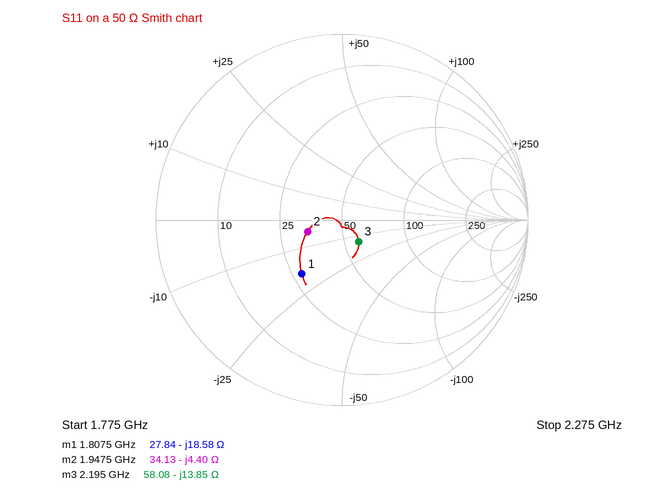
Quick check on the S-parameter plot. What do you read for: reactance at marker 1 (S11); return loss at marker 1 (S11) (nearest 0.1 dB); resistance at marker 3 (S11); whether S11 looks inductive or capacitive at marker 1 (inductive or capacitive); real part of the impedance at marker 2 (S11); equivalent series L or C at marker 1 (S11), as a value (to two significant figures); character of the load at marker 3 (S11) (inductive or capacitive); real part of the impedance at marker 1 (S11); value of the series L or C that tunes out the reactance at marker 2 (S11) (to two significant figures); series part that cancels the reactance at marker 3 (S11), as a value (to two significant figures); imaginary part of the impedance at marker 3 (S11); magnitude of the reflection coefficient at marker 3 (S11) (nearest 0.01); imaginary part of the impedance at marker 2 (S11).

-18.58 Ω
8.8 dB
58.08 Ω
capacitive
34.13 Ω
4.7 pF
capacitive
27.84 Ω
360 pH
1.0 nH
-13.85 Ω
0.15
-4.40 Ω
